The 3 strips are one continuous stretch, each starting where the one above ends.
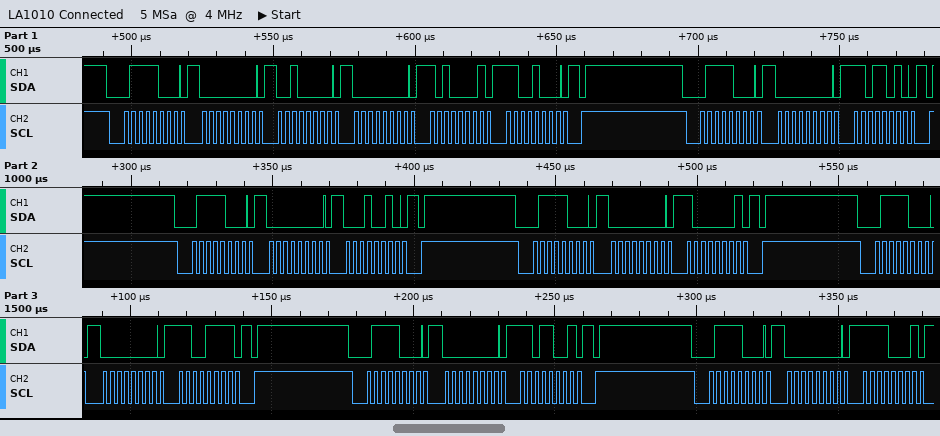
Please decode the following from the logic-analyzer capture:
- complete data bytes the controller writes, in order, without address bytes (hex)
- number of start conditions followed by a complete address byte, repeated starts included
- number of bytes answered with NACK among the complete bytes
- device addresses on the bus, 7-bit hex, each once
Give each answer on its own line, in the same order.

00 20 00 A1 C8 00 DA 00 12 00 81 00 CF 00 D9 00 F1
7
0
0x3C
